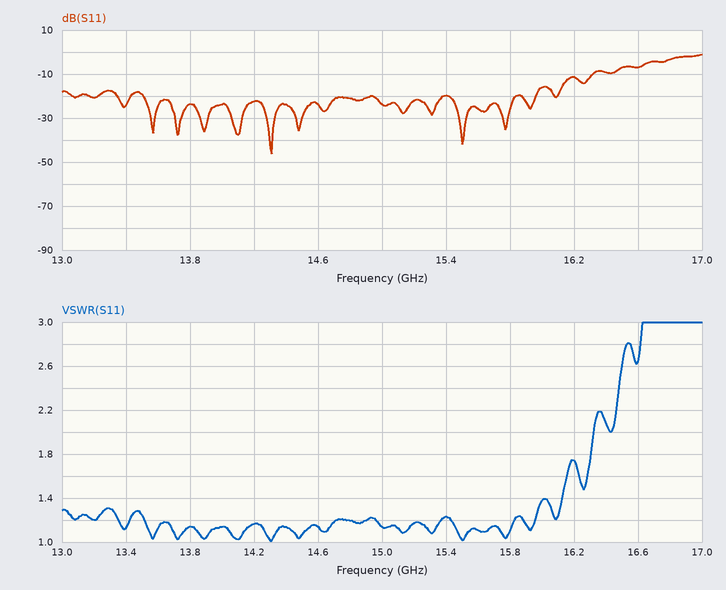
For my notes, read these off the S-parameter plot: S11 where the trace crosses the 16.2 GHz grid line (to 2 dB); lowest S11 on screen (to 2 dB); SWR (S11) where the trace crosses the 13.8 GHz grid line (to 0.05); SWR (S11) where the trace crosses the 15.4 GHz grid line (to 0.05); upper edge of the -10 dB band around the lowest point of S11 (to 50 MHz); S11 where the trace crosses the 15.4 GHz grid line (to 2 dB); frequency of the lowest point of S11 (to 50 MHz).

-12 dB
-46 dB
1.15
1.25
16.30 GHz
-20 dB
14.30 GHz
